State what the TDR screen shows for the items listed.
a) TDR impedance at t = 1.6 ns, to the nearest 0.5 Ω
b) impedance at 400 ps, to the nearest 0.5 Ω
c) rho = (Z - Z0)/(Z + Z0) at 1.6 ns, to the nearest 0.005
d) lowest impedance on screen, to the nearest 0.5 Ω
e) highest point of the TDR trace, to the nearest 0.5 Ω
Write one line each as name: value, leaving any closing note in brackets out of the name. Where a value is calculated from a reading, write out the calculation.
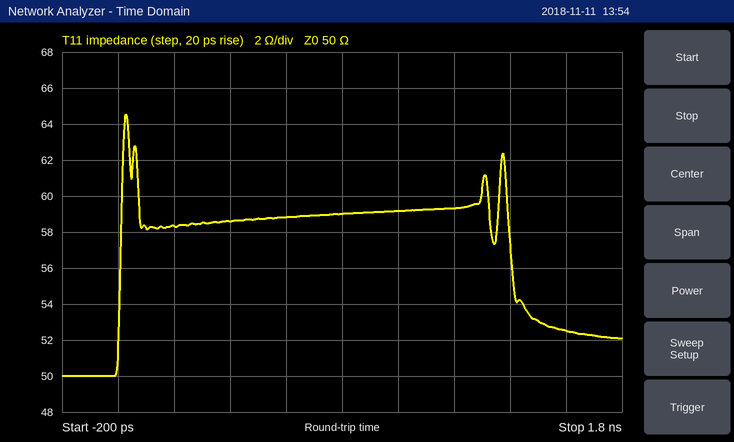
TDR impedance at t = 1.6 ns, to the nearest 0.5 Ω: 52.5 Ω
impedance at 400 ps, to the nearest 0.5 Ω: 58.5 Ω
rho = (Z - Z0)/(Z + Z0) at 1.6 ns, to the nearest 0.005: (52.5 − 50)/(52.5 + 50) ≈ +0.0244, so +0.025 to the nearest 0.005
lowest impedance on screen, to the nearest 0.5 Ω: 50.0 Ω
highest point of the TDR trace, to the nearest 0.5 Ω: 64.5 Ω
